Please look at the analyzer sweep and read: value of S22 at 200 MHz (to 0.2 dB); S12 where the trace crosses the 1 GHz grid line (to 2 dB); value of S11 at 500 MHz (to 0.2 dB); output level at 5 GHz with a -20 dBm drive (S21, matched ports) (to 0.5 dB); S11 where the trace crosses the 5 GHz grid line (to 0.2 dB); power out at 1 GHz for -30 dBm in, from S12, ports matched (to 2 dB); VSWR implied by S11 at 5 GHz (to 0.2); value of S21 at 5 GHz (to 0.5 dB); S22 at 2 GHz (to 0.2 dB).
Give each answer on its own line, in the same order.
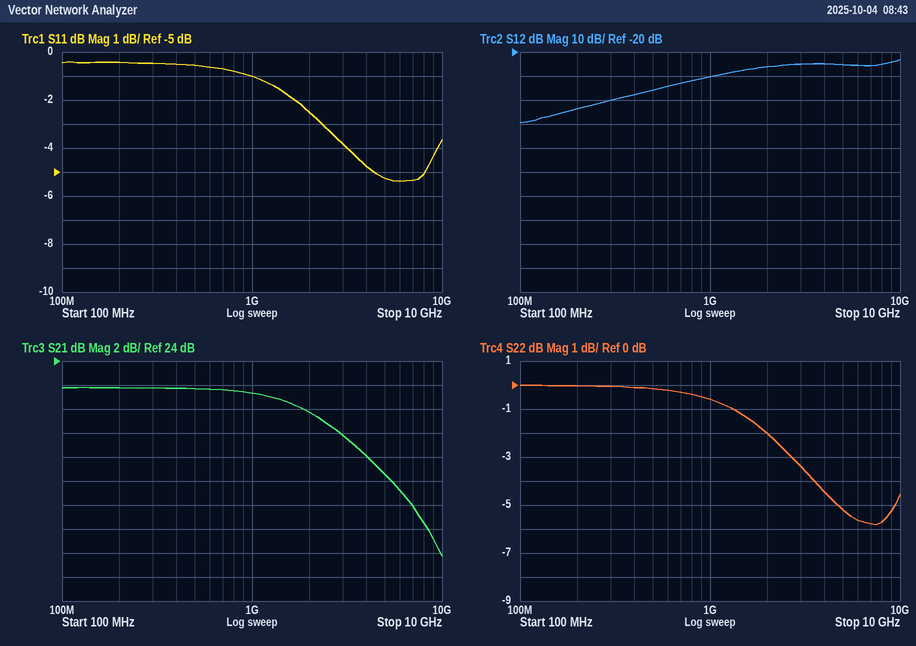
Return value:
0.0 dB
-30 dB
-0.6 dB
-5.5 dBm
-5.2 dB
-60 dBm
3.4
14.5 dB
-2.0 dB
